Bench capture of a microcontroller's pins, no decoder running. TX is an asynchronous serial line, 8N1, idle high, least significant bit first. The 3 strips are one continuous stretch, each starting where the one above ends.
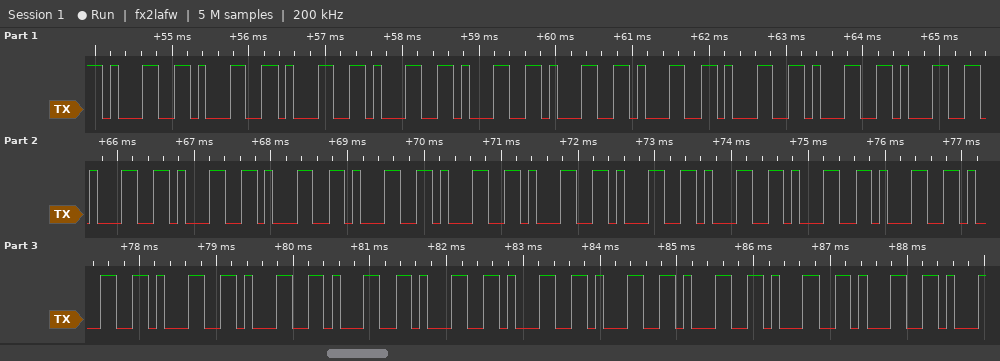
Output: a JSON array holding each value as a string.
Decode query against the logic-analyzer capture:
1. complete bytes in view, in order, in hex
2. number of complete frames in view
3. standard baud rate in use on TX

["31 31 31 31 31 31 31 31 31 31 31 31 31 31 31 31 31 31 31 31 31 31 31 31 31 31 31 31 31 31", "30", "9600 baud"]
